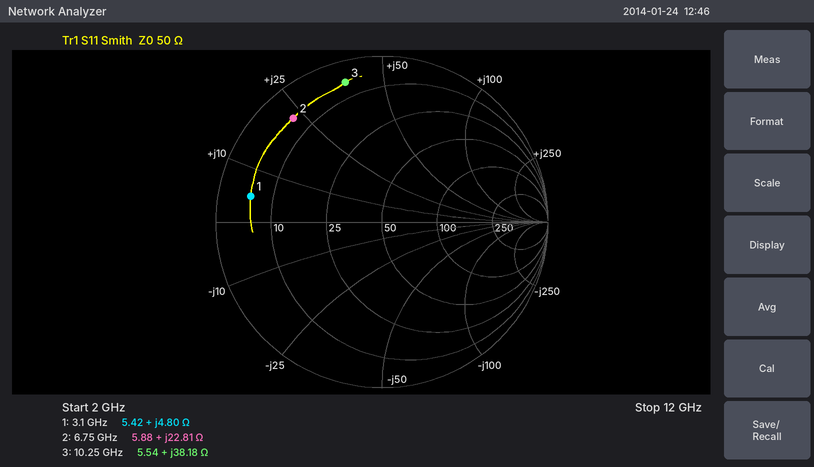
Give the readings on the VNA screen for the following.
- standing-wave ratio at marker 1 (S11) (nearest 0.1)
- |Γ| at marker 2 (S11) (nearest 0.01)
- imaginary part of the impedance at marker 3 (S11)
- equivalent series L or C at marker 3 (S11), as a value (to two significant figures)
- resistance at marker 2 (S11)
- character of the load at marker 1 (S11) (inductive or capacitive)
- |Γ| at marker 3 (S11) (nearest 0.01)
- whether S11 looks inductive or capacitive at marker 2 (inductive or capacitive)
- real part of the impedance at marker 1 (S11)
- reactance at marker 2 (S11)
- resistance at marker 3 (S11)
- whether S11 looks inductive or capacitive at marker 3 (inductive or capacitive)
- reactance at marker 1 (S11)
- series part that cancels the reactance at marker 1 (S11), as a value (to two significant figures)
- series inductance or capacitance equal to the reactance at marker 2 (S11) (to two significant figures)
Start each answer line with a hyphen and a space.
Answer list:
- 9.3
- 0.82
- +38.18 Ω
- 590 pH
- 5.88 Ω
- inductive
- 0.87
- inductive
- 5.42 Ω
- +22.81 Ω
- 5.54 Ω
- inductive
- +4.80 Ω
- 11 pF
- 540 pH
